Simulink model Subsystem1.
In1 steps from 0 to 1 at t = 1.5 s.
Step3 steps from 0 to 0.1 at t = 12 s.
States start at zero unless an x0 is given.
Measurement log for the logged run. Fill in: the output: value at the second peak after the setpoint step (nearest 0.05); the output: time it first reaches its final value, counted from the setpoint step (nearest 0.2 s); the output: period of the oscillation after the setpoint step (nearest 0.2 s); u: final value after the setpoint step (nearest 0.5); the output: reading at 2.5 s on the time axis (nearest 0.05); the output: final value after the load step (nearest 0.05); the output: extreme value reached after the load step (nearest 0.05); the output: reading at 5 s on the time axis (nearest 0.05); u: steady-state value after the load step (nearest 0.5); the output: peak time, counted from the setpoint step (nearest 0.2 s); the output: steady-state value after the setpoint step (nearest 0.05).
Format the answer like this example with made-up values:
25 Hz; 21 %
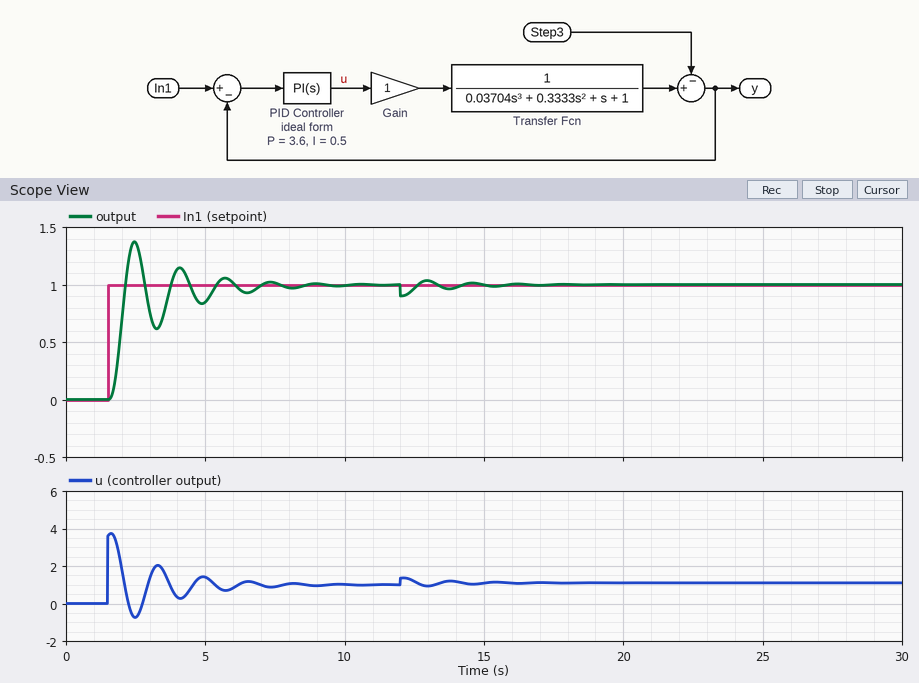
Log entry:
1.15; 0.6 s; 1.6 s; 1.0; 1.35; 1.00; 0.90; 0.85; 1.0; 1.0 s; 1.00
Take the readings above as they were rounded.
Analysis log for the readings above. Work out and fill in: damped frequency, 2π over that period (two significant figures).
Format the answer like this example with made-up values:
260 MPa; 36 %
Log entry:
3.9 rad/s
